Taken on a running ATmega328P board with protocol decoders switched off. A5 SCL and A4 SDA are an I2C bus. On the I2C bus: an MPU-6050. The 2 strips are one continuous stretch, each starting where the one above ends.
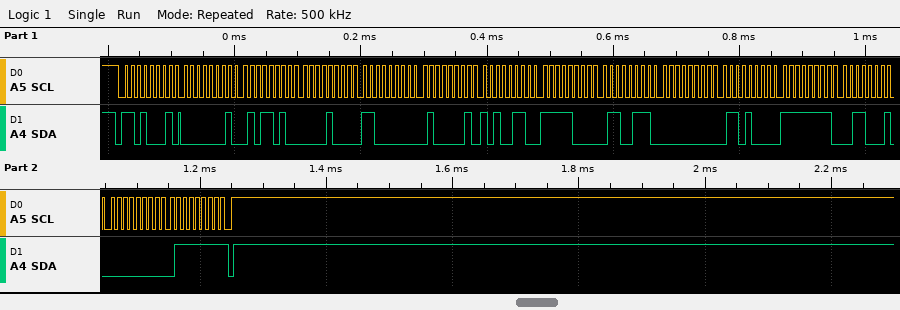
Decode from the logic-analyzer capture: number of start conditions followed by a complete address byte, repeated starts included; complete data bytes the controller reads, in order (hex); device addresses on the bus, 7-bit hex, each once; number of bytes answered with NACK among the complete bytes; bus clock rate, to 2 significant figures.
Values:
1
01 5A 08 C0 41 A6 F8 67 00 68 FF 31 00 7F
0x68
1
100 kHz
